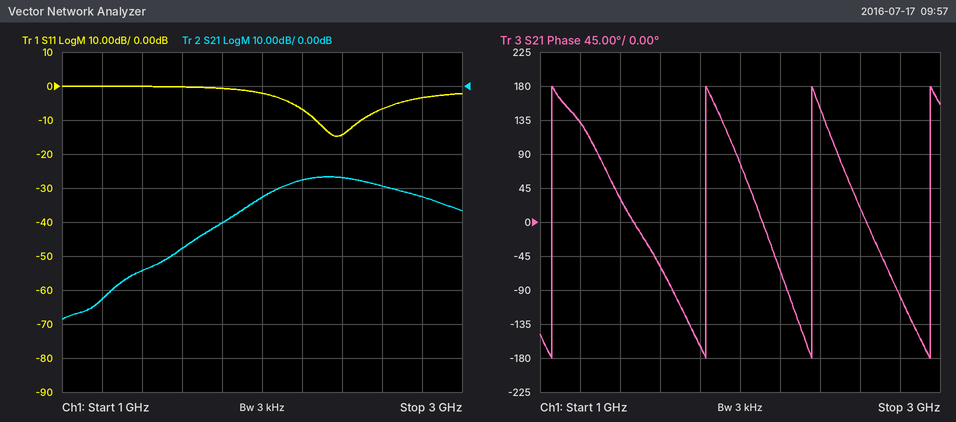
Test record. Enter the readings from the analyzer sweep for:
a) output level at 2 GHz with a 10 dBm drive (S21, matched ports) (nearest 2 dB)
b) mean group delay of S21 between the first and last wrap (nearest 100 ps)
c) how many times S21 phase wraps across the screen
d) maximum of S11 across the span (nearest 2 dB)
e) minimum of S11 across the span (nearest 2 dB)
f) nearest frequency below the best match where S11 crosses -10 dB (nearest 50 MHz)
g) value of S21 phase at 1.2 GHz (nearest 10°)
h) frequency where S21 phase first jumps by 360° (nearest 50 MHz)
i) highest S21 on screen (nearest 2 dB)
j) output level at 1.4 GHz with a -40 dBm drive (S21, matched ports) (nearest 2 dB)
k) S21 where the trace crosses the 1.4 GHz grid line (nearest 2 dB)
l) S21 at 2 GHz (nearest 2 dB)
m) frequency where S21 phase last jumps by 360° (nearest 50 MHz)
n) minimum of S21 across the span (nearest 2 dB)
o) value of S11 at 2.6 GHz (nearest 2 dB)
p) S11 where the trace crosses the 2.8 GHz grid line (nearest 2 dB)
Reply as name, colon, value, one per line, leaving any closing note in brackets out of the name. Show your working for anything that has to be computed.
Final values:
output level at 2 GHz with a 10 dBm drive (S21, matched ports): 10 dBm + (-32 dB) = -22 dBm
mean group delay of S21 between the first and last wrap: 3 cycles / (2.95 GHz − 1.05 GHz) ≈ 1.6 ns
how many times S21 phase wraps across the screen: 4
maximum of S11 across the span: 0 dB
minimum of S11 across the span: -14 dB
nearest frequency below the best match where S11 crosses -10 dB: 2.25 GHz
value of S21 phase at 1.2 GHz: 130°
frequency where S21 phase first jumps by 360°: 1.05 GHz
highest S21 on screen: -26 dB
output level at 1.4 GHz with a -40 dBm drive (S21, matched ports): -40 dBm + (-54 dB) = -94 dBm
S21 where the trace crosses the 1.4 GHz grid line: -54 dB
S21 at 2 GHz: -32 dB
frequency where S21 phase last jumps by 360°: 2.95 GHz
minimum of S21 across the span: -68 dB
value of S11 at 2.6 GHz: -6 dB
S11 where the trace crosses the 2.8 GHz grid line: -4 dB
